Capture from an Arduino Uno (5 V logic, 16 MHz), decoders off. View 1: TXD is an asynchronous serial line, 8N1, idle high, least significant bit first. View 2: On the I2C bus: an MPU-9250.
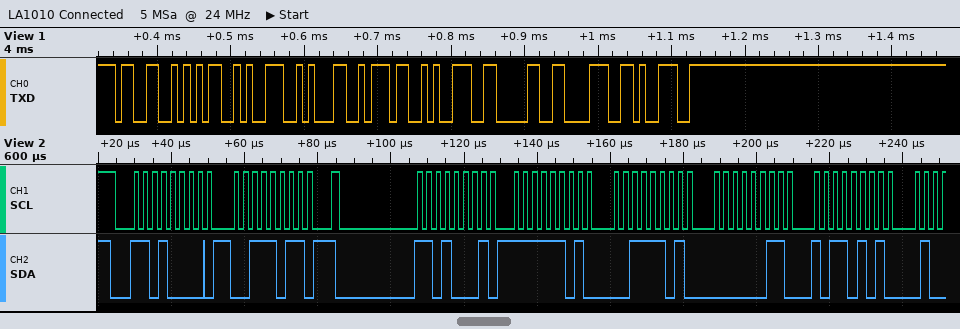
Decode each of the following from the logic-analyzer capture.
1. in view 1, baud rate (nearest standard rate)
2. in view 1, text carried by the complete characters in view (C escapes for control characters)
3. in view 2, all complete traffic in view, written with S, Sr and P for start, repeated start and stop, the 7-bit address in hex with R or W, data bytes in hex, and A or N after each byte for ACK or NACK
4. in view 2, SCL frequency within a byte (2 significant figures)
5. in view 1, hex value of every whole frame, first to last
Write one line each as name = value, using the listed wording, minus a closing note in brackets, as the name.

in view 1, baud rate = 115200 baud
in view 1, text carried by the complete characters in view = "359179089"
in view 2, all complete traffic in view, written with S, Sr and P for start, repeated start and stop, the 7-bit address in hex with R or W, data bytes in hex, and A or N after each byte for ACK or NACK = S 68W A 3B A Sr 68R A FD A 3D A 03 A B5 A
in view 2, SCL frequency within a byte = 400 kHz
in view 1, hex value of every whole frame, first to last = 0x33 0x35 0x39 0x31 0x37 0x39 0x30 0x38 0x39
